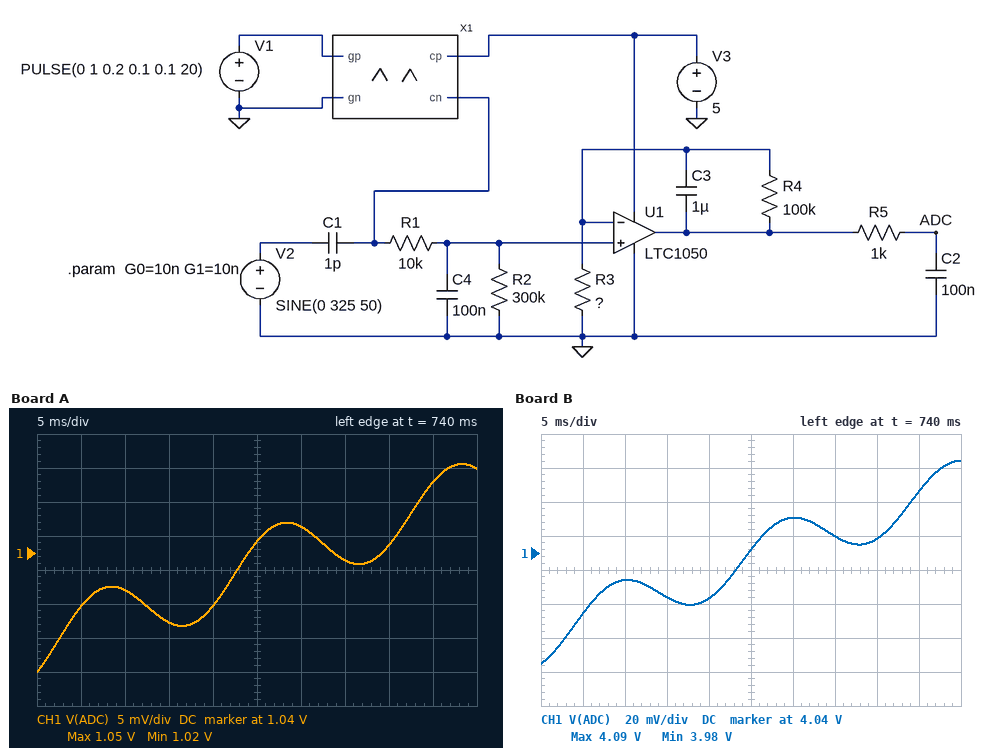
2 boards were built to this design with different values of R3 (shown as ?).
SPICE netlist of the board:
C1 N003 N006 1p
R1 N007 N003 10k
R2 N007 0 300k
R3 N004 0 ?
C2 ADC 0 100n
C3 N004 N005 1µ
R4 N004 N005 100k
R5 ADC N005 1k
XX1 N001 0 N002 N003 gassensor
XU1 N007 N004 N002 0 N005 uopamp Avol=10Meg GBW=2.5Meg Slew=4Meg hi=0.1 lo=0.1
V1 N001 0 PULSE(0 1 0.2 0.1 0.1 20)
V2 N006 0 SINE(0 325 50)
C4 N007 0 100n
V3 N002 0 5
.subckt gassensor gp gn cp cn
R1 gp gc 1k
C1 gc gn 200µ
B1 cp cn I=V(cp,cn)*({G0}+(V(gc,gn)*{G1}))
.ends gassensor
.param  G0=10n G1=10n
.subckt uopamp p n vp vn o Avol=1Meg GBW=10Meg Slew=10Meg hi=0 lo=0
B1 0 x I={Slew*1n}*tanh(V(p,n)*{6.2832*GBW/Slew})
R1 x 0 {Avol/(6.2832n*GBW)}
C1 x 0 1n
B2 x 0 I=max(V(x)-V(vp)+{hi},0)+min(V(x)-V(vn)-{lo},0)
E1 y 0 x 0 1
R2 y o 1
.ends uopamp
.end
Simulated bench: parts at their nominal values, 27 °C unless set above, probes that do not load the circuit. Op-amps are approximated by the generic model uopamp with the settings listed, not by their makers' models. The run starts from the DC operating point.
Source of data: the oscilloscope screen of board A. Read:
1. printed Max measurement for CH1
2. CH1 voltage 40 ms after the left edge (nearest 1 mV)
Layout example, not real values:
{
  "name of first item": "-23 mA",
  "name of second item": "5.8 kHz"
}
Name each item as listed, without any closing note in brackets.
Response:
{
  "printed Max measurement for CH1": "1.05 V",
  "CH1 voltage 40 ms after the left edge": "1.041 V"
}
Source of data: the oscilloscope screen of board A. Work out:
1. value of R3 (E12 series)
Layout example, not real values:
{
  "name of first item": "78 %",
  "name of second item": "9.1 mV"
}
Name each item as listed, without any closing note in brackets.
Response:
{
  "value of R3": "2.7 kΩ"
}
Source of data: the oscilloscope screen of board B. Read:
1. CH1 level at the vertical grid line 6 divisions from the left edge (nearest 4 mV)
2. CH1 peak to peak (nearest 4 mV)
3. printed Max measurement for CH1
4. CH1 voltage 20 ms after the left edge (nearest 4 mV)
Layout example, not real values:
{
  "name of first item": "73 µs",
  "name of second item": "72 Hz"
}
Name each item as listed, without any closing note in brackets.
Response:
{
  "CH1 level at the vertical grid line 6 divisions from the left edge": "4.060 V",
  "CH1 peak to peak": "120 mV",
  "printed Max measurement for CH1": "4.09 V",
  "CH1 voltage 20 ms after the left edge": "4.012 V"
}
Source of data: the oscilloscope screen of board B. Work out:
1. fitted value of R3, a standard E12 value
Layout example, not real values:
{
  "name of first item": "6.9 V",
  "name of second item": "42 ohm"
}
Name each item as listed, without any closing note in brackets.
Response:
{
  "fitted value of R3, a standard E12 value": "680 Ω"
}
